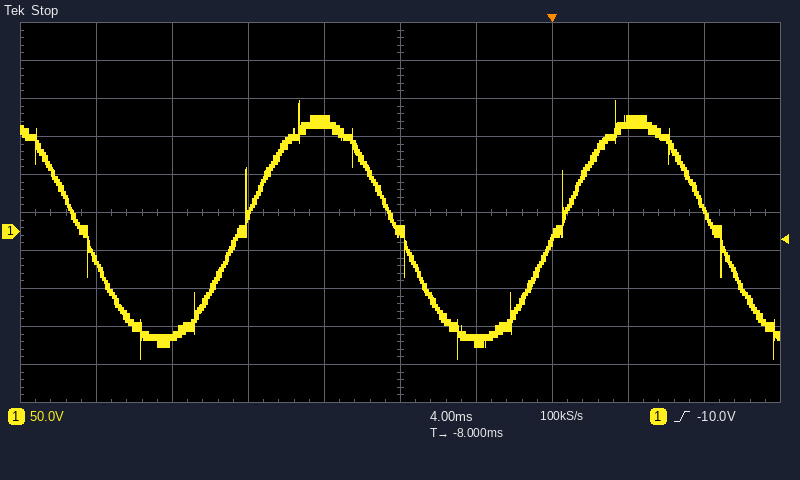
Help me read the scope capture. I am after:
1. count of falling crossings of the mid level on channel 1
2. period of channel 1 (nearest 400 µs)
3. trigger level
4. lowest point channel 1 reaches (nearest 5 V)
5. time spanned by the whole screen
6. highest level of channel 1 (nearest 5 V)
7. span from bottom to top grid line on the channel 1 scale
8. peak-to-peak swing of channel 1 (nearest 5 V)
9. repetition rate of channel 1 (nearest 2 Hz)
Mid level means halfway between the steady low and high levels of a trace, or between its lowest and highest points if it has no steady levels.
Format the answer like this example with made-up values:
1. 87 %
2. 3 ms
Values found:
1. 3
2. 16.8 ms
3. -10.0 V
4. -170 V
5. 40 ms
6. 170 V
7. 500 V
8. 340 V
9. 60 Hz
